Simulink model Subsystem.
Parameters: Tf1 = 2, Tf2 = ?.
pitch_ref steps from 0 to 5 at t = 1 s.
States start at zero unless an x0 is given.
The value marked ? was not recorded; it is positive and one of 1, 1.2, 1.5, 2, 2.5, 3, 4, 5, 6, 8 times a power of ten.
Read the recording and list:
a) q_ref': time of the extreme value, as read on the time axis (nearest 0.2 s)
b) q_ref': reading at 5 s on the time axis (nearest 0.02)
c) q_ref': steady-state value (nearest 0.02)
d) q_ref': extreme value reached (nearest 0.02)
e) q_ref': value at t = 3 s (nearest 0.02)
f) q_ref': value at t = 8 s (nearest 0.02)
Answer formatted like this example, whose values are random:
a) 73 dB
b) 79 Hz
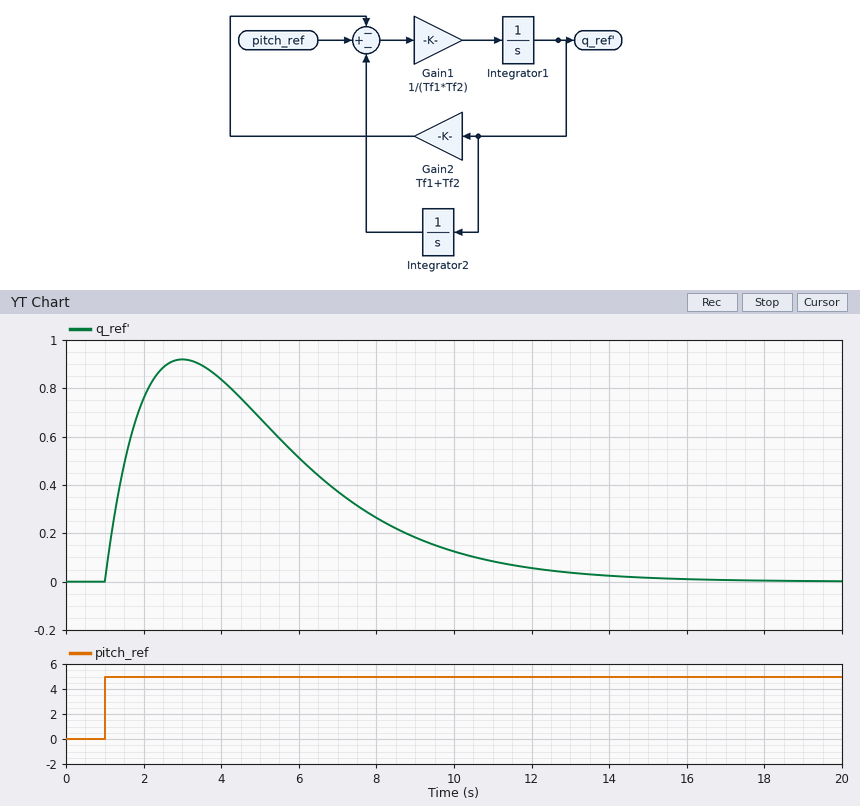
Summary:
a) 3.0 s
b) 0.68
c) 0.00
d) 0.92
e) 0.92
f) 0.26
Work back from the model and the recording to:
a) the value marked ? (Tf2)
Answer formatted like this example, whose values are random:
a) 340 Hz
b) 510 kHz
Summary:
a) 2
